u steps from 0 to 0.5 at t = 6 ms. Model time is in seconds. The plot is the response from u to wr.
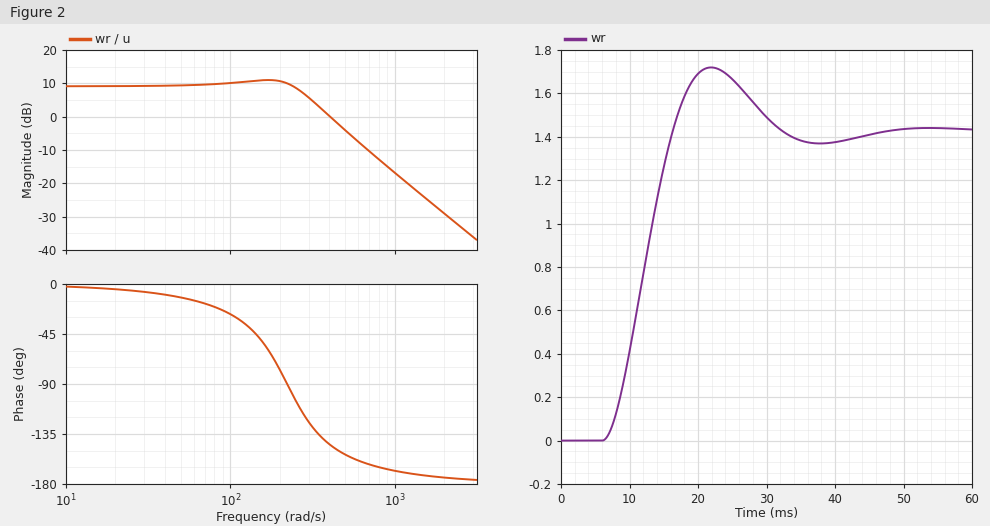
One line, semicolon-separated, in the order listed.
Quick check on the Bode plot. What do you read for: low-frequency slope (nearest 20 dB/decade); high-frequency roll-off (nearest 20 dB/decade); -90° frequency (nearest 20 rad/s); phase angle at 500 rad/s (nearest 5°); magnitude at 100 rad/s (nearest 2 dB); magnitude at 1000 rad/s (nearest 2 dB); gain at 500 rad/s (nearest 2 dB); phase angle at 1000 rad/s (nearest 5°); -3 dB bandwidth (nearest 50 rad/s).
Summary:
0 dB/decade; -40 dB/decade; 220 rad/s; -155°; 10 dB; -16 dB; -4 dB; -170°; 300 rad/s
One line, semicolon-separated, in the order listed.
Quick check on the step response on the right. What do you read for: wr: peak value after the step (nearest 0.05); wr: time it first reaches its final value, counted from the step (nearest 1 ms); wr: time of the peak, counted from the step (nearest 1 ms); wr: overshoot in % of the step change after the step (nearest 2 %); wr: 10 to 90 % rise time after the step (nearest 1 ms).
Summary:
1.70; 10 ms; 16 ms; 20 %; 7 ms
